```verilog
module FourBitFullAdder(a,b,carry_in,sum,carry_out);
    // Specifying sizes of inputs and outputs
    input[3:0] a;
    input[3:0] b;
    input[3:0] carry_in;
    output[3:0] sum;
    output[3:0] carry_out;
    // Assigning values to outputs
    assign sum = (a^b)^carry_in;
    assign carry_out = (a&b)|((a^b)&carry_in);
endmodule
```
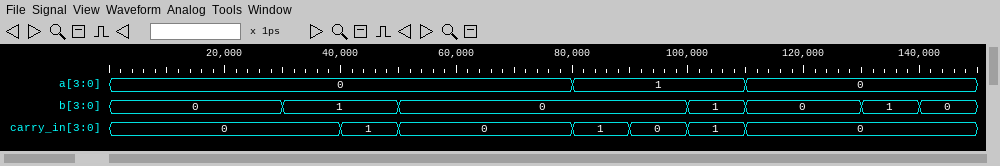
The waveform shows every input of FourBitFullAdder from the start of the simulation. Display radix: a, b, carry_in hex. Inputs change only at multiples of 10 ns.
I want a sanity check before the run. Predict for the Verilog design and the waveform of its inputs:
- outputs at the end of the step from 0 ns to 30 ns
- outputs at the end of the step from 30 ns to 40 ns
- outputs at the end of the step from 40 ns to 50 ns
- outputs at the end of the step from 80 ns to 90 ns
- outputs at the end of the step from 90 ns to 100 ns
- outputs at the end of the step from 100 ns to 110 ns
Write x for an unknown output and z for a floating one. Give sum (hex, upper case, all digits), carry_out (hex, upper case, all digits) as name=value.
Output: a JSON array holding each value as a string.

["sum=0, carry_out=0", "sum=1, carry_out=0", "sum=0, carry_out=1", "sum=0, carry_out=1", "sum=1, carry_out=0", "sum=1, carry_out=1"]
